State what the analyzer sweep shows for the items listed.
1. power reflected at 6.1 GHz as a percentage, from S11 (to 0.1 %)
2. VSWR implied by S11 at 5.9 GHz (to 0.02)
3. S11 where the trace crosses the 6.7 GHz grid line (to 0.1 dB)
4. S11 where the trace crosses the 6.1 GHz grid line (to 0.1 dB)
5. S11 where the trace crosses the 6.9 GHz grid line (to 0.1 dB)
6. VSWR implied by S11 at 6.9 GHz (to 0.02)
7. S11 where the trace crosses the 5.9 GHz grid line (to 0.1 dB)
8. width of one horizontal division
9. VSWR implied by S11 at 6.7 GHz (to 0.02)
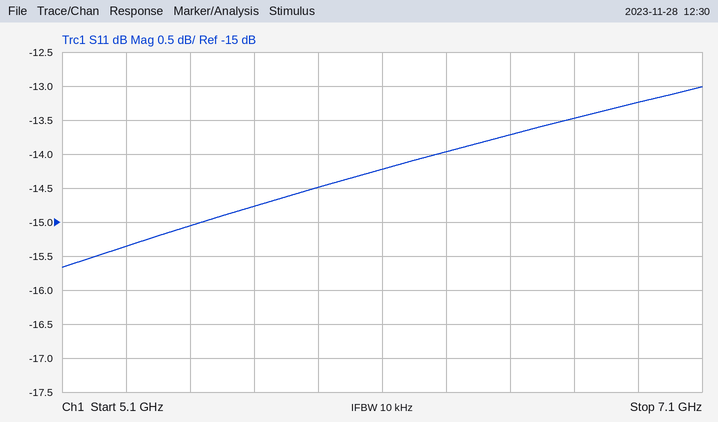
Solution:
3.8 %
1.46
-13.5 dB
-14.2 dB
-13.2 dB
1.56
-14.5 dB
200 MHz
1.54
